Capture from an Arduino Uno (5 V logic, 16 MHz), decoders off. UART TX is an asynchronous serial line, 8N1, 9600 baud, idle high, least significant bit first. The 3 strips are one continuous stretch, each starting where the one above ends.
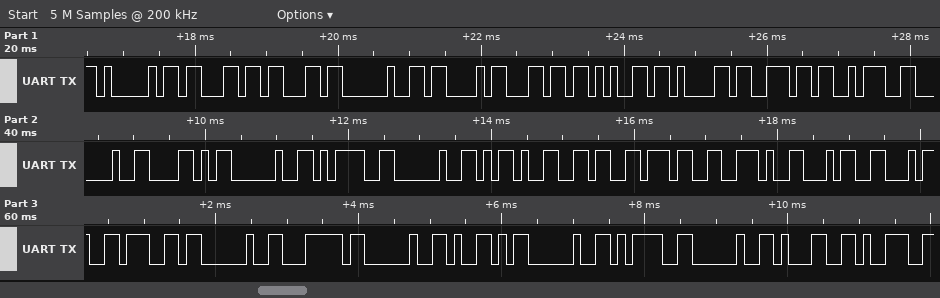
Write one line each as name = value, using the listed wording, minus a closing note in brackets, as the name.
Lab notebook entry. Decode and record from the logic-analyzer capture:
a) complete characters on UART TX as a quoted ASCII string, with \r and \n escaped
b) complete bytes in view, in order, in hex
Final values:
complete characters on UART TX as a quoted ASCII string, with \r and \n escaped = "Acc Clean: X = -67.44g | Y = 19"
complete bytes in view, in order, in hex = 41 63 63 20 43 6C 65 61 6E 3A 20 58 20 3D 20 2D 36 37 2E 34 34 67 20 7C 20 59 20 3D 20 31 39
